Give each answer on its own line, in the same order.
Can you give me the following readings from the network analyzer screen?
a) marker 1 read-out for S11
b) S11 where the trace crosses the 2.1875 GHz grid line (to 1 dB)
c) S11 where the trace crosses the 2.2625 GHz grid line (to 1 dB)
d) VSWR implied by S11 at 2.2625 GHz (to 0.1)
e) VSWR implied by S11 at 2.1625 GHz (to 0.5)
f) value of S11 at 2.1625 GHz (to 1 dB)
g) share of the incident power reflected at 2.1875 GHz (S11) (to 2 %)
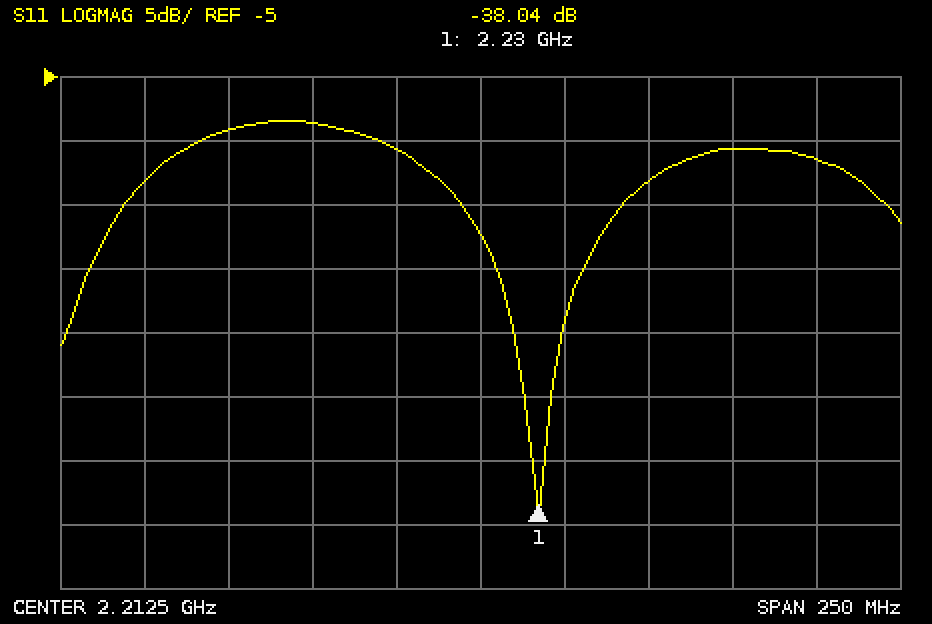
-38.04 dB
-11 dB
-13 dB
1.6
2.0
-9 dB
8 %
